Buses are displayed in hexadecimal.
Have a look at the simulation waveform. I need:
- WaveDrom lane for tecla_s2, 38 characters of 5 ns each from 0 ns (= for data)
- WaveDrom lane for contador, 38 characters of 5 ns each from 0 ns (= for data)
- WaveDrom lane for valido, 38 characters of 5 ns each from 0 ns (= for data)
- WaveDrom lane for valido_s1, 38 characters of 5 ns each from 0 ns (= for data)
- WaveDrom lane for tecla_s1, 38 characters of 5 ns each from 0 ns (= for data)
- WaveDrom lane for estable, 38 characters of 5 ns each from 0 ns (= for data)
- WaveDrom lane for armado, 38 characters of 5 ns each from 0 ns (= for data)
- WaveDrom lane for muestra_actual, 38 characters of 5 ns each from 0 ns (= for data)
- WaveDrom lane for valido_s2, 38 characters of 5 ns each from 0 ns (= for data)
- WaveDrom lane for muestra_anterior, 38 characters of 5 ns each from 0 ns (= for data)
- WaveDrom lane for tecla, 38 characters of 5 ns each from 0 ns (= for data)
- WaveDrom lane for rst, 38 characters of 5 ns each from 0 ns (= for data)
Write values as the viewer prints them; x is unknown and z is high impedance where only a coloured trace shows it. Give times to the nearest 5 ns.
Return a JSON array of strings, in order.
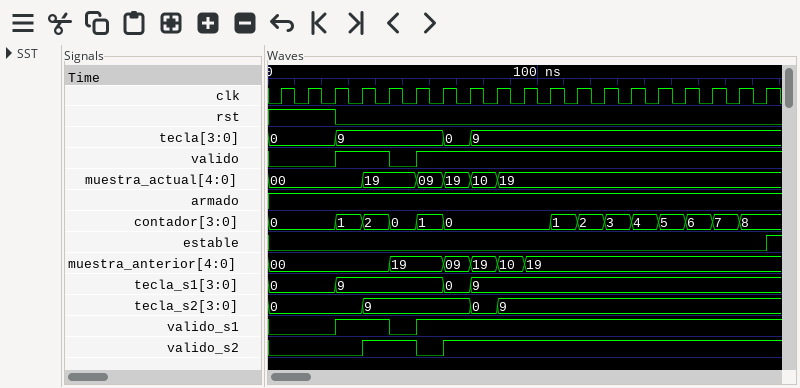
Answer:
["{name: 'tecla_s2', wave: '=......=.......=.=....................', data: '0 9 0 9'}", "{name: 'contador', wave: '=....=.=.=.=.=.......=.=.=.=.=.=.=.=..', data: '0 1 2 0 1 0 1 2 3 4 5 6 7 8'}", "{name: 'valido', wave: '0....1...0.1..........................'}", "{name: 'valido_s1', wave: '0....1...0.1..........................'}", "{name: 'tecla_s1', wave: '=....=.......=.=......................', data: '0 9 0 9'}", "{name: 'estable', wave: '0....................................1'}", "{name: 'armado', wave: '1.....................................'}", "{name: 'muestra_actual', wave: '=......=...=.=.=.=....................', data: '00 19 09 19 10 19'}", "{name: 'valido_s2', wave: '0......1...0.1........................'}", "{name: 'muestra_anterior', wave: '=........=...=.=.=.=..................', data: '00 19 09 19 10 19'}", "{name: 'tecla', wave: '=....=.......=.=......................', data: '0 9 0 9'}", "{name: 'rst', wave: '1....0................................'}"]
